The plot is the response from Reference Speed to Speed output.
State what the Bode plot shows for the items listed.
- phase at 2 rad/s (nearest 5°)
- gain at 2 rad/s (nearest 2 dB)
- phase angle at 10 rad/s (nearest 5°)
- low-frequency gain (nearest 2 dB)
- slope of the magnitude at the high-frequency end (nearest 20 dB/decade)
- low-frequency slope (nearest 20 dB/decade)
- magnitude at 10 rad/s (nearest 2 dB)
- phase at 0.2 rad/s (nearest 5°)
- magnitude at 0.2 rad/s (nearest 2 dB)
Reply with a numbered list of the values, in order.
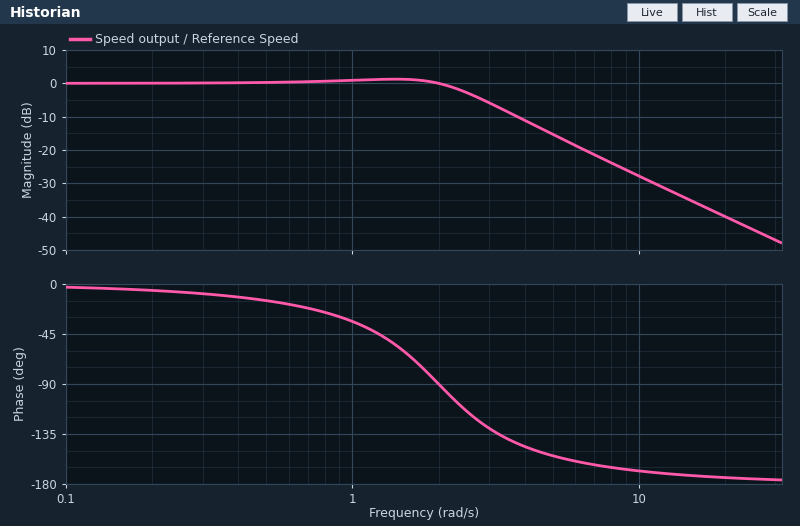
1. -90°
2. 0 dB
3. -170°
4. 0 dB
5. -40 dB/decade
6. 0 dB/decade
7. -28 dB
8. -5°
9. 0 dB
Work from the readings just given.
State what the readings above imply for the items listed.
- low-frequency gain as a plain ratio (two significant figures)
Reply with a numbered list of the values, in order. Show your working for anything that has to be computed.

1. 10^(0 / 20) = 1.0
